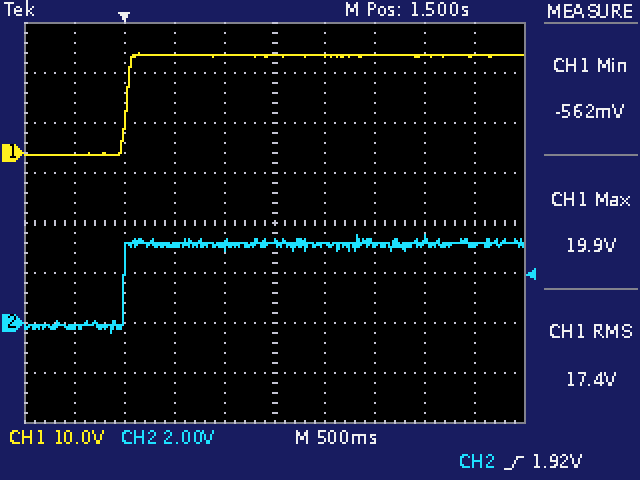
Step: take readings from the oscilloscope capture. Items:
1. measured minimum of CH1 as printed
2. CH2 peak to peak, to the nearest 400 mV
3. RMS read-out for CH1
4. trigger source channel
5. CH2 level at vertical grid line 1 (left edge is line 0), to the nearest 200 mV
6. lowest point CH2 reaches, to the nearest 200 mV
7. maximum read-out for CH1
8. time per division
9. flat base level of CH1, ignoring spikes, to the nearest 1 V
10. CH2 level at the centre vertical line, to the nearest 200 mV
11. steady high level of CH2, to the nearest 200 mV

-562 mV
4.0 V
17.4 V
CH2
-200 mV
-400 mV
19.9 V
500 ms
0 V
3.2 V
3.2 V
